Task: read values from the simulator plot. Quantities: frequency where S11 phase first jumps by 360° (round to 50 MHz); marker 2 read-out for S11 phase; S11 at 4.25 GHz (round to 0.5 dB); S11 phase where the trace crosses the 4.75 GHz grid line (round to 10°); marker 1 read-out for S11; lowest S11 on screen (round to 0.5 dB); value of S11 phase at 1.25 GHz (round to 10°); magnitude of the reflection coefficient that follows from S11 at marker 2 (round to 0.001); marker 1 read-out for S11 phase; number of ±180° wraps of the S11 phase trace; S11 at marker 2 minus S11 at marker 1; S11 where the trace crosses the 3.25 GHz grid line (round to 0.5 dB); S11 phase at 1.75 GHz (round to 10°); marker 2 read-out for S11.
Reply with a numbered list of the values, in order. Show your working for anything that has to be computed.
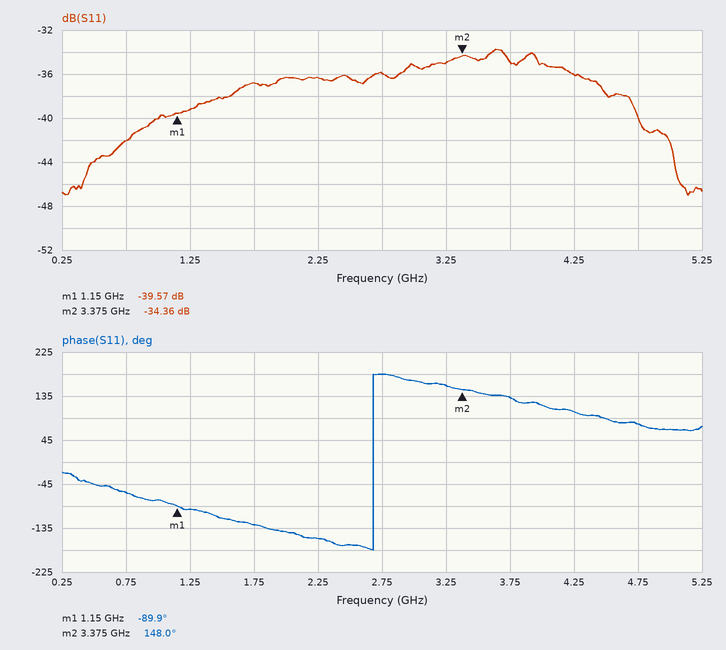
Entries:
1. 2.70 GHz
2. 148.0°
3. -36.0 dB
4. 80°
5. -39.57 dB
6. -47.0 dB
7. -100°
8. 10^(-34.36/20) ≈ 0.019
9. -89.9°
10. 1
11. -34.36 − (-39.57) = 5.21 dB
12. -35.0 dB
13. -130°
14. -34.36 dB
